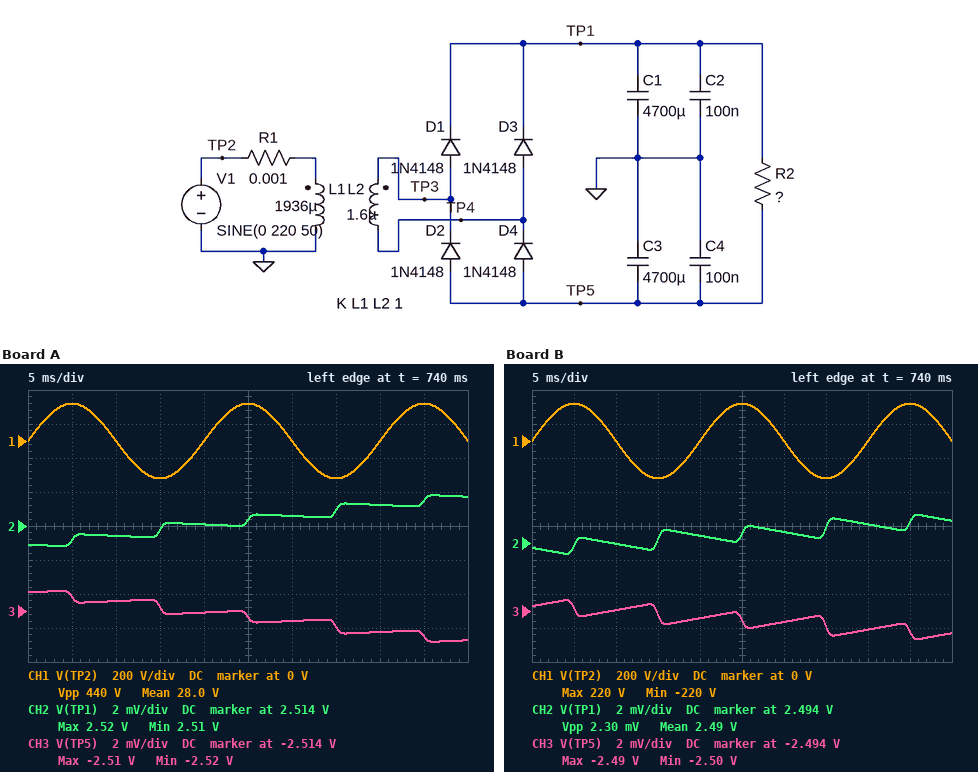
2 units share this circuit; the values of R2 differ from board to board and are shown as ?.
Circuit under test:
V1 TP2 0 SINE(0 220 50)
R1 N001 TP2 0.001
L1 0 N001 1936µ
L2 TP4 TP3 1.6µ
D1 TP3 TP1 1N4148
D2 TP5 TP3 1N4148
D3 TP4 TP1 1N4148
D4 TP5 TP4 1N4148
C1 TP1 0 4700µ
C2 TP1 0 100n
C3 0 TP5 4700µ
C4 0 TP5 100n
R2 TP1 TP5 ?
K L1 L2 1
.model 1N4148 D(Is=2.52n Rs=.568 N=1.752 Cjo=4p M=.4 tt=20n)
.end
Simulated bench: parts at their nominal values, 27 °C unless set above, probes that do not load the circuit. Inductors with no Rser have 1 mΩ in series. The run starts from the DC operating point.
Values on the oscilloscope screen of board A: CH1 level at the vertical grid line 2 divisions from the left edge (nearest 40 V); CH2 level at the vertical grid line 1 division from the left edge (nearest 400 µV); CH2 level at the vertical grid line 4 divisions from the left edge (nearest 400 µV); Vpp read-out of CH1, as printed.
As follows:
0 V
2.5132 V
2.5140 V
440 V
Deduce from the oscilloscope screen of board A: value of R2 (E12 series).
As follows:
47 kΩ
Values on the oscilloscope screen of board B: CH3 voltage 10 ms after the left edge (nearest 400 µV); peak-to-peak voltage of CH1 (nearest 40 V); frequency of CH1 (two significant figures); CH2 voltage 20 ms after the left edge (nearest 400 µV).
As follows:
-2.4940 V
440 V
50 Hz
2.4944 V
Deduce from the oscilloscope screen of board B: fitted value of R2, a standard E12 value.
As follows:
12 kΩ
